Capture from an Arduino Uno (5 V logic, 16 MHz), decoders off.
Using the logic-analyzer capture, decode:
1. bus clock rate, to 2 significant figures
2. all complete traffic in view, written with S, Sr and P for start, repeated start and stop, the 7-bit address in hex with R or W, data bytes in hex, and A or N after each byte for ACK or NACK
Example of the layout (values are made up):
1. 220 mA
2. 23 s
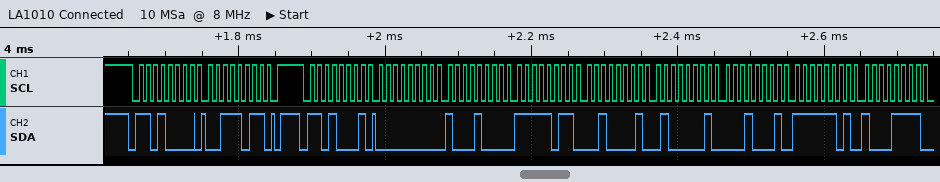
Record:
1. 100 kHz
2. S 68W A 3B A P S 68R A 00 A 88 A FB A 21 A 41 A 11 A FD A 8F A
